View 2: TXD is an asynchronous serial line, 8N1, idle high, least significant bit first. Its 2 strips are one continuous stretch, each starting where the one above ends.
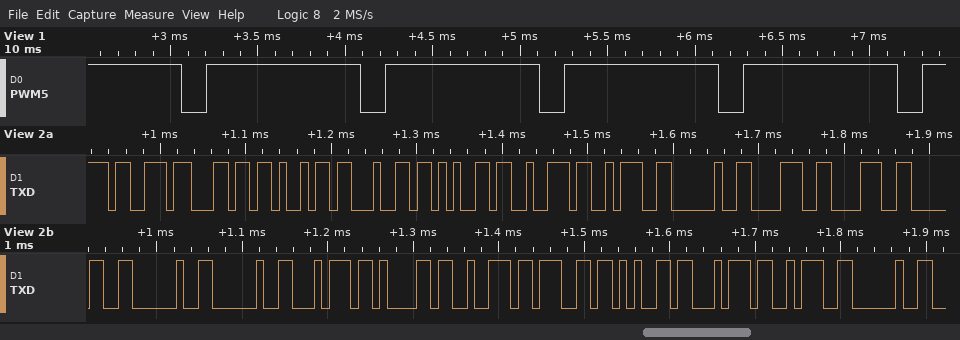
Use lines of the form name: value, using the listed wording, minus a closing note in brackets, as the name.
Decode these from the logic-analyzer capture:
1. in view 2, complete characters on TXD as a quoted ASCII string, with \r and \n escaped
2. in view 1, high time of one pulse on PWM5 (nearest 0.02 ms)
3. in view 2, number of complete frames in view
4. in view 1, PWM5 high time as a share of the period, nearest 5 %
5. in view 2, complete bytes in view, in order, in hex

in view 2, complete characters on TXD as a quoted ASCII string, with \r and \n escaped: "slider: 880  target: "
in view 1, high time of one pulse on PWM5: 0.88 ms
in view 2, number of complete frames in view: 21
in view 1, PWM5 high time as a share of the period, nearest 5 %: 85 %
in view 2, complete bytes in view, in order, in hex: 73 6C 69 64 65 72 3A 20 38 38 30 20 20 74 61 72 67 65 74 3A 20
